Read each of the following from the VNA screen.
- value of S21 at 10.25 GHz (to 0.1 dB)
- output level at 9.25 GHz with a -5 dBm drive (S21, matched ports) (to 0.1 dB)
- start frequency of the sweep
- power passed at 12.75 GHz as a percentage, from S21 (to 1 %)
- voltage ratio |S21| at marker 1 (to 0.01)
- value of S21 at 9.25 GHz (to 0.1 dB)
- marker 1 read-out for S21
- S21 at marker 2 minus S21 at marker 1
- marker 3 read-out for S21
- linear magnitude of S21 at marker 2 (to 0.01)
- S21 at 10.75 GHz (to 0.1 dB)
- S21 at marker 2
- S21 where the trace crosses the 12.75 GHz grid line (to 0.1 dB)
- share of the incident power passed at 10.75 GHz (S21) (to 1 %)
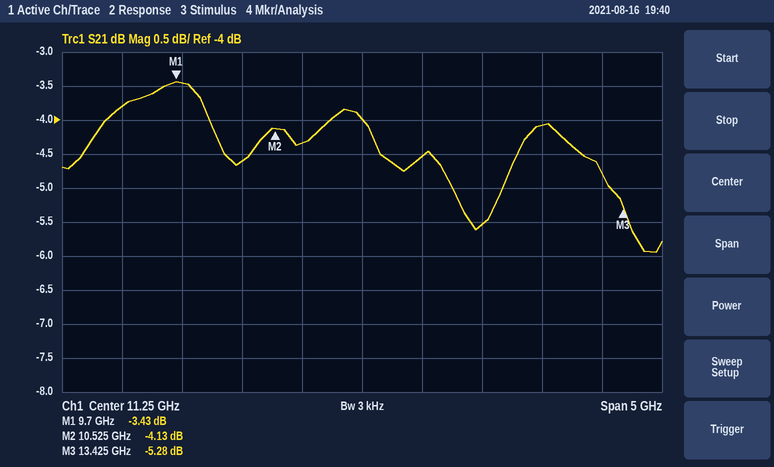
-4.6 dB
-8.8 dBm
8.75 GHz
39 %
0.67
-3.8 dB
-3.43 dB
-0.70 dB
-5.28 dB
0.62
-4.3 dB
-4.13 dB
-4.1 dB
37 %
